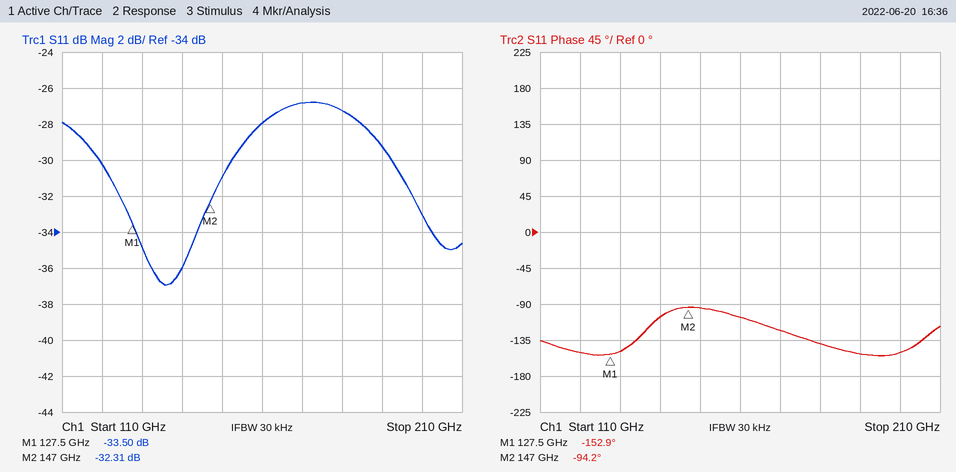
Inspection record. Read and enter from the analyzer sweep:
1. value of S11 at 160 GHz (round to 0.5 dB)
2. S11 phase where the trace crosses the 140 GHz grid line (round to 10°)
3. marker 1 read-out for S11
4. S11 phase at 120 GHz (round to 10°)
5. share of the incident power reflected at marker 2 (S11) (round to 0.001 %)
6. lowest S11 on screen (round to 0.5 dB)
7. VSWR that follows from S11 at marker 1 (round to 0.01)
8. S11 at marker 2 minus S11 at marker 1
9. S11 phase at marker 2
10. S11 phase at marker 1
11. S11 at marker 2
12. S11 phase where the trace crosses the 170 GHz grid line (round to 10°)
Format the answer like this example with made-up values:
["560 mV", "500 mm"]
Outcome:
["-28.0 dB", "-110°", "-33.50 dB", "-150°", "0.059 %", "-37.0 dB", "1.04", "1.19 dB", "-94.2°", "-152.9°", "-32.31 dB", "-120°"]
